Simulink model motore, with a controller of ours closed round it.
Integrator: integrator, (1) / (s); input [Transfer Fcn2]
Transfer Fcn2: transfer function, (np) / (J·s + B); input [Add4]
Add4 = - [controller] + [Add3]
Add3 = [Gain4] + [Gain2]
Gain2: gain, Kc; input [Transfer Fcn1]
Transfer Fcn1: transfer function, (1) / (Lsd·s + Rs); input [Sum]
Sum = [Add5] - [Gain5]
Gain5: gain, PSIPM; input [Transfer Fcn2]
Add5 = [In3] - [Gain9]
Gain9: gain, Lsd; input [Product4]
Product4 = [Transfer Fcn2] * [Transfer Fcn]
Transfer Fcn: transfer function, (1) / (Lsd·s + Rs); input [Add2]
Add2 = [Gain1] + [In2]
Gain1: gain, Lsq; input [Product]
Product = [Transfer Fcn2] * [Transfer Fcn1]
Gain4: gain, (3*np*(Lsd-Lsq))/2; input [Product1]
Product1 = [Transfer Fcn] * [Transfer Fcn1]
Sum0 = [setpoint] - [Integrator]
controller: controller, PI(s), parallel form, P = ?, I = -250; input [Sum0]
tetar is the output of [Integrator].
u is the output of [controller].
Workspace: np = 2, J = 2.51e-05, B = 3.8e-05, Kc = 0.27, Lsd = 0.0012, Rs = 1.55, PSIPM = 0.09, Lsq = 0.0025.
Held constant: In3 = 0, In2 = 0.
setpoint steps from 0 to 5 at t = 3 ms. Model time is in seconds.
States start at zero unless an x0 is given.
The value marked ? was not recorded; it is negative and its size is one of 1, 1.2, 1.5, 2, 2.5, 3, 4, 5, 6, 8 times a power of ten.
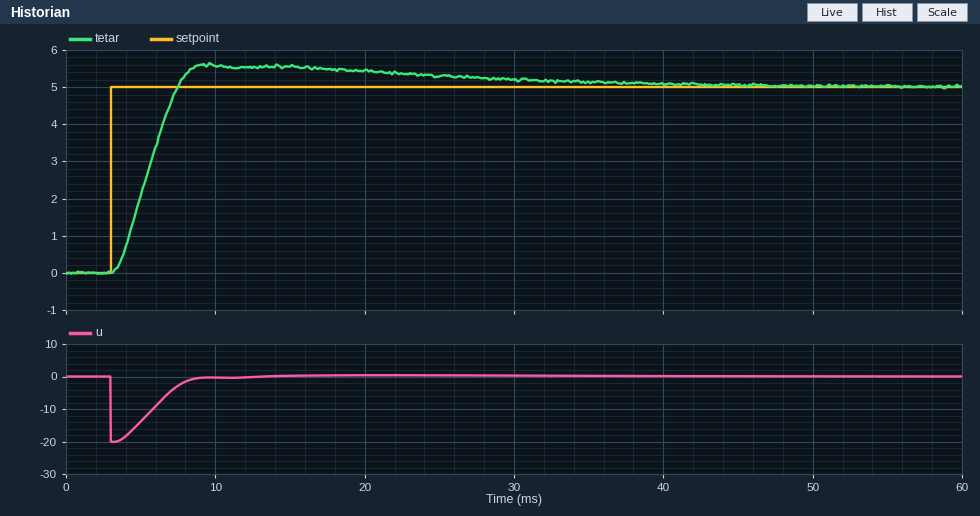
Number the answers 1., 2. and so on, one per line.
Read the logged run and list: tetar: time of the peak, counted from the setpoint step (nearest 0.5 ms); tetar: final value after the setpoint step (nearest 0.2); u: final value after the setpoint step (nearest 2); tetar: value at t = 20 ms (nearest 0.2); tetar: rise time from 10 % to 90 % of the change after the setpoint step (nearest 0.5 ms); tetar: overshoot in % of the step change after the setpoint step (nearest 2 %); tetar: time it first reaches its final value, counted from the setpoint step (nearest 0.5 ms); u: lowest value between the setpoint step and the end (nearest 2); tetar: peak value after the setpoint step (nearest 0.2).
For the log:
1. 6.5 ms
2. 5.0
3. 0
4. 5.4
5. 3.0 ms
6. 12 %
7. 4.5 ms
8. -20
9. 5.6
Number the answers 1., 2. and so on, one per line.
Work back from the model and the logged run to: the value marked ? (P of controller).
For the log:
1. -4
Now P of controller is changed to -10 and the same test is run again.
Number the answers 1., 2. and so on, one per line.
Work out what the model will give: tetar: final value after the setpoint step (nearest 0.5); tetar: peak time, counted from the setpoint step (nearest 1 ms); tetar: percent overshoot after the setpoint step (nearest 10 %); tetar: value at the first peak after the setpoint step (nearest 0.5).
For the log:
1. 5.0
2. 4 ms
3. 70 %
4. 8.5
